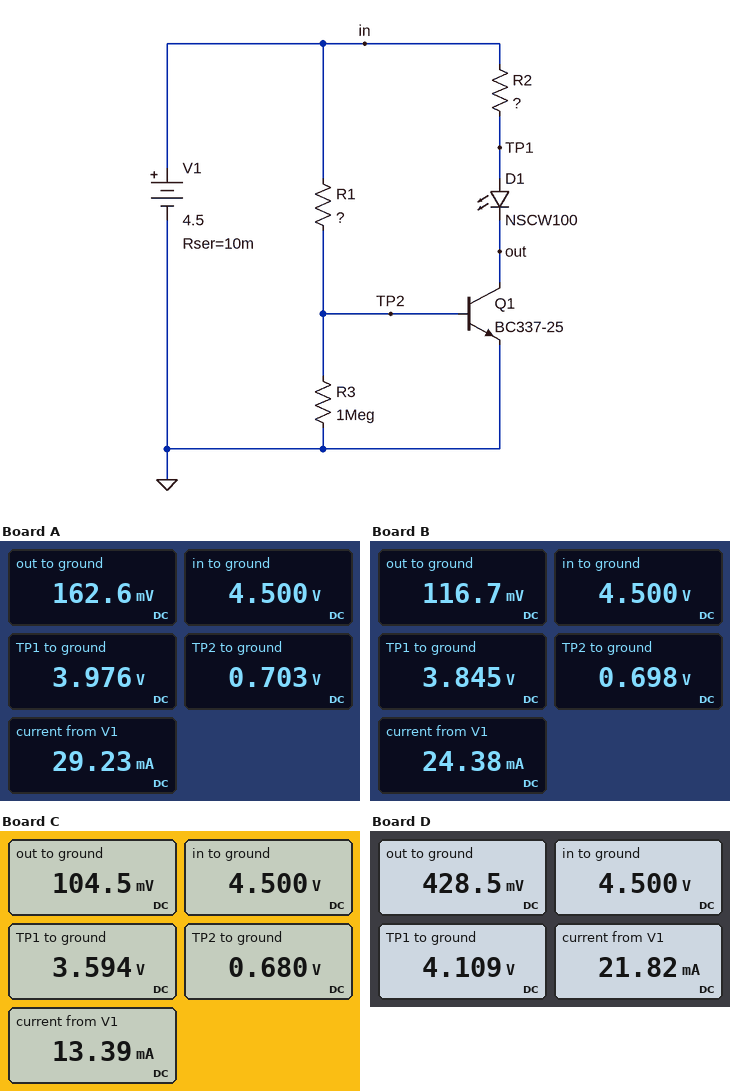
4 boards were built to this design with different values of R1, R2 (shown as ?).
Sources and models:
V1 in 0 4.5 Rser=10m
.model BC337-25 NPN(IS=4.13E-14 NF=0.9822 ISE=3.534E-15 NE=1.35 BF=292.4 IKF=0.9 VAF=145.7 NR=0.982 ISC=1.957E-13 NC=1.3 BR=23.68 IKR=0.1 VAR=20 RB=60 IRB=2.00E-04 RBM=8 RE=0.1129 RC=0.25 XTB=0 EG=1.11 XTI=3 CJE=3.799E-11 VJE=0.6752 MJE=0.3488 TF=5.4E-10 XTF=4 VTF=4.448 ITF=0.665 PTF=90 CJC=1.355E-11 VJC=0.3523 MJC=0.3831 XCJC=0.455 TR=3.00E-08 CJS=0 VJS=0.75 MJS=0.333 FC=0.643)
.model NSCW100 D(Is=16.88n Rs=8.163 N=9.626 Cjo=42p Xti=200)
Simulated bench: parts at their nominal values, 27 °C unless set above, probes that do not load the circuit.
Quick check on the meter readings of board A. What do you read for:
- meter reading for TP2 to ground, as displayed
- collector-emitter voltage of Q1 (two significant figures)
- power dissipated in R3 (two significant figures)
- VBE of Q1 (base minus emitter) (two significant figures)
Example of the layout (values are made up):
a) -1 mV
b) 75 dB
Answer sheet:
a) 0.703 V
b) 160 mV
c) 490 nW
d) 700 mV
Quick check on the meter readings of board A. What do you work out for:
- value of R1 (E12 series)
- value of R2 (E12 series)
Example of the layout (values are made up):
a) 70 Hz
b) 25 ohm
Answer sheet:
a) 33 kΩ
b) 18 Ω
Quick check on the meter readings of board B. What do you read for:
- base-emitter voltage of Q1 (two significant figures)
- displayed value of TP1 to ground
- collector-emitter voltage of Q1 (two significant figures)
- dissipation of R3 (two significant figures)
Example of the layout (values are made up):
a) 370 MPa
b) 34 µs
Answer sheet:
a) 700 mV
b) 3.845 V
c) 120 mV
d) 490 nW
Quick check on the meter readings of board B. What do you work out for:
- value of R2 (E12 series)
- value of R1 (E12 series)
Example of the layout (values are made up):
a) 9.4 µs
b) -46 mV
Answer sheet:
a) 27 Ω
b) 33 kΩ
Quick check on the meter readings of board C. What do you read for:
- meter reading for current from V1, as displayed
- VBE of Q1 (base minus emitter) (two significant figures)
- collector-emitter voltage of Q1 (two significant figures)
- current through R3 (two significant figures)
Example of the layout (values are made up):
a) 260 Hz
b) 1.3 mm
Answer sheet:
a) 13.39 mA
b) 680 mV
c) 100 mV
d) 680 nA
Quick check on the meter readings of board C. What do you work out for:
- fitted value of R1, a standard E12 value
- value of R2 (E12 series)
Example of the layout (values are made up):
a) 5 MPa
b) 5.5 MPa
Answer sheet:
a) 56 kΩ
b) 68 Ω
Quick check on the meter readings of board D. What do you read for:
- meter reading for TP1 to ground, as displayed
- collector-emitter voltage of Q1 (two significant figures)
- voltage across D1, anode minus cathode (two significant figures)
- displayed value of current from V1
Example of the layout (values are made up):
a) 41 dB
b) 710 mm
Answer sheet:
a) 4.109 V
b) 430 mV
c) 3.7 V
d) 21.82 mA
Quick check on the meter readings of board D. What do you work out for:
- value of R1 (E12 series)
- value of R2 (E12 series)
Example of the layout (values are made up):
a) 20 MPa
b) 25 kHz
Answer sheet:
a) 47 kΩ
b) 18 Ω
